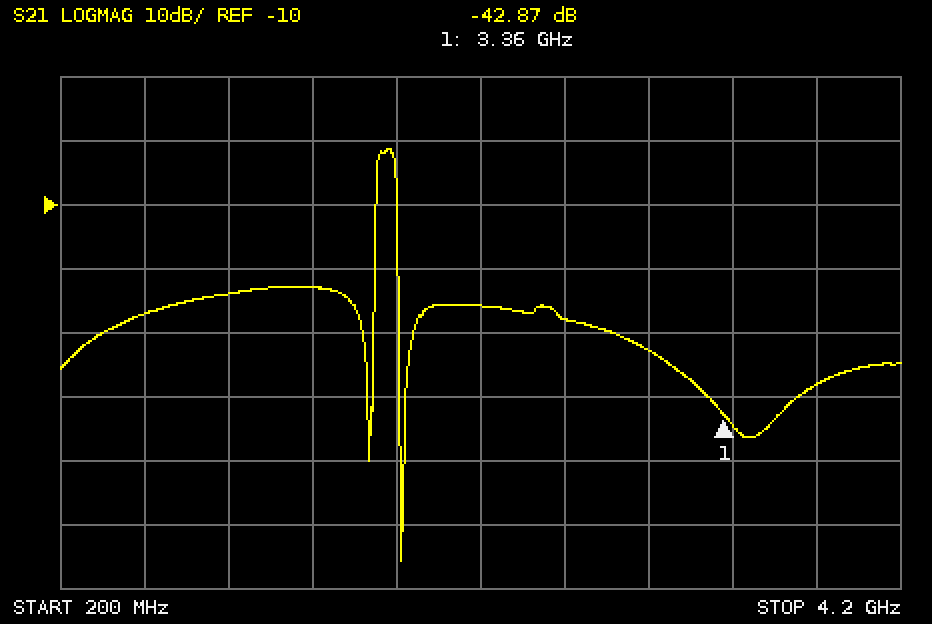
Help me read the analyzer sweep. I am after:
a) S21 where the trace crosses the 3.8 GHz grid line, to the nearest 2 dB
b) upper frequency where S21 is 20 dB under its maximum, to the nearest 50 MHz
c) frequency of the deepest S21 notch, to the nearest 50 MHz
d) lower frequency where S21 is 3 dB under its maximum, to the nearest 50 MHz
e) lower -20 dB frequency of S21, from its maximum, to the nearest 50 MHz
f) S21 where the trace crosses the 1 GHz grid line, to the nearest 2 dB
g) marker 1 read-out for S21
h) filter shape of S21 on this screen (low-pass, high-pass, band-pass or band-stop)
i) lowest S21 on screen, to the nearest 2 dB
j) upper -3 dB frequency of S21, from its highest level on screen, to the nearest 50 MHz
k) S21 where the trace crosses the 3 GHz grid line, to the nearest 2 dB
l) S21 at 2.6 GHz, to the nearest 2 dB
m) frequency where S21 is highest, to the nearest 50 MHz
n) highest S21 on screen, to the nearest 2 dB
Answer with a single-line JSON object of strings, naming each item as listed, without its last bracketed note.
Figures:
{"S21 where the trace crosses the 3.8 GHz grid line, to the nearest 2 dB": "-38 dB", "upper frequency where S21 is 20 dB under its maximum, to the nearest 50 MHz": "1.80 GHz", "frequency of the deepest S21 notch, to the nearest 50 MHz": "1.80 GHz", "lower frequency where S21 is 3 dB under its maximum, to the nearest 50 MHz": "1.70 GHz", "lower -20 dB frequency of S21, from its maximum, to the nearest 50 MHz": "1.70 GHz", "S21 where the trace crosses the 1 GHz grid line, to the nearest 2 dB": "-24 dB", "marker 1 read-out for S21": "-42.87 dB", "filter shape of S21 on this screen": "band-pass", "lowest S21 on screen, to the nearest 2 dB": "-66 dB", "upper -3 dB frequency of S21, from its highest level on screen, to the nearest 50 MHz": "1.80 GHz", "S21 where the trace crosses the 3 GHz grid line, to the nearest 2 dB": "-32 dB", "S21 at 2.6 GHz, to the nearest 2 dB": "-28 dB", "frequency where S21 is highest, to the nearest 50 MHz": "1.75 GHz", "highest S21 on screen, to the nearest 2 dB": "-2 dB"}
